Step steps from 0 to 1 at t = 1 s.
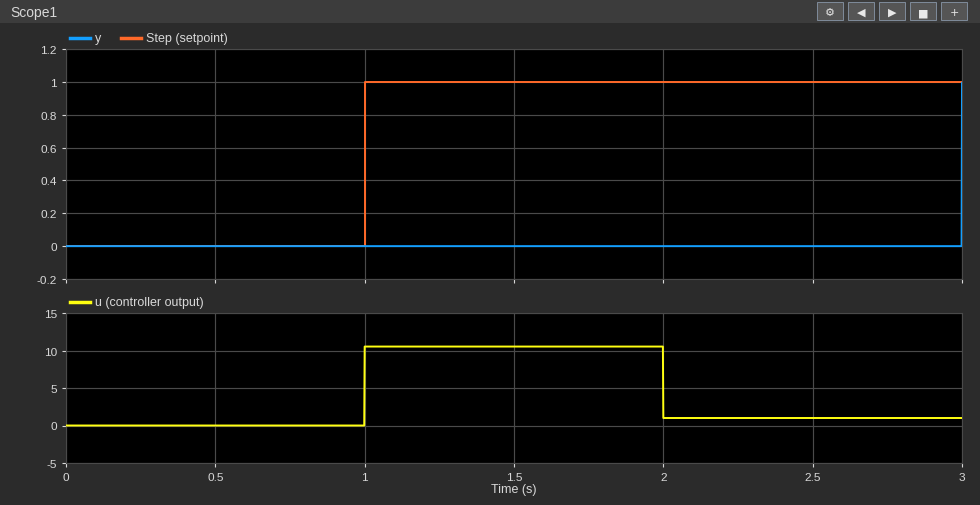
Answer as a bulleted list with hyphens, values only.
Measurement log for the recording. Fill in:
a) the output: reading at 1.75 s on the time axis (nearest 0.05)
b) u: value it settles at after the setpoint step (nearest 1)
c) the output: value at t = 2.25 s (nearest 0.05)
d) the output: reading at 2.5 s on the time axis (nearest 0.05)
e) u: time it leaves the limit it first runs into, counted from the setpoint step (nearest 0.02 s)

- 0.00
- 1
- 0.00
- 0.00
- 1.00 s
